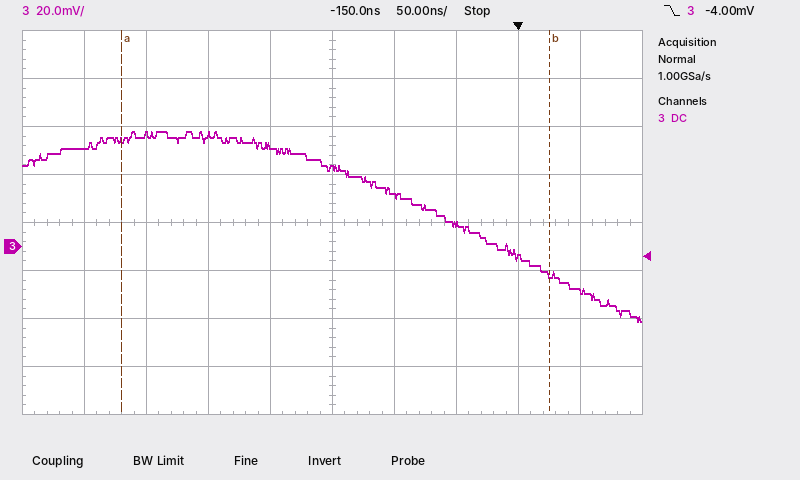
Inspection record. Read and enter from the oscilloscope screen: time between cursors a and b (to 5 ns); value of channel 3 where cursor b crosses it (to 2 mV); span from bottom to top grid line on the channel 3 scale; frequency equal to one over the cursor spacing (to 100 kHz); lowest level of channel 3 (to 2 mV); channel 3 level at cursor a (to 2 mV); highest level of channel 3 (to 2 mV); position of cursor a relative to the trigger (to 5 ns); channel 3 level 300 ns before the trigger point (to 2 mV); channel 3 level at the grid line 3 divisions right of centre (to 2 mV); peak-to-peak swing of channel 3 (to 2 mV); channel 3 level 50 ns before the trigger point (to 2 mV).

345 ns
-12 mV
160 mV
2.9 MHz
-32 mV
44 mV
48 mV
-320 ns
46 mV
-4 mV
80 mV
10 mV
